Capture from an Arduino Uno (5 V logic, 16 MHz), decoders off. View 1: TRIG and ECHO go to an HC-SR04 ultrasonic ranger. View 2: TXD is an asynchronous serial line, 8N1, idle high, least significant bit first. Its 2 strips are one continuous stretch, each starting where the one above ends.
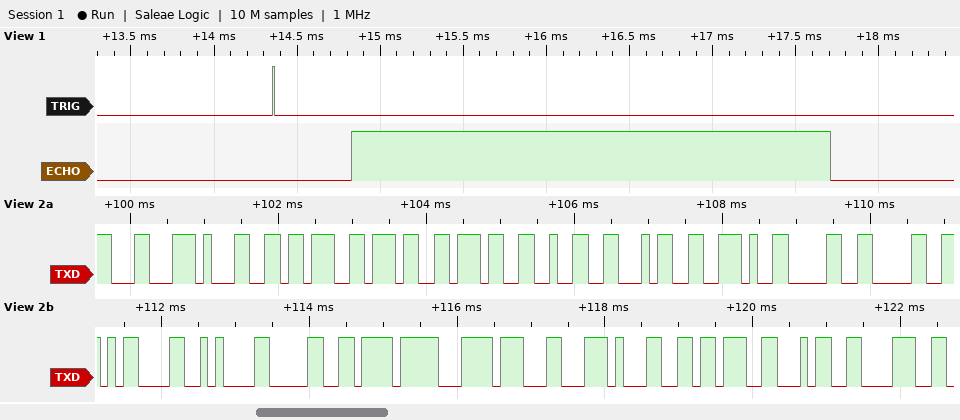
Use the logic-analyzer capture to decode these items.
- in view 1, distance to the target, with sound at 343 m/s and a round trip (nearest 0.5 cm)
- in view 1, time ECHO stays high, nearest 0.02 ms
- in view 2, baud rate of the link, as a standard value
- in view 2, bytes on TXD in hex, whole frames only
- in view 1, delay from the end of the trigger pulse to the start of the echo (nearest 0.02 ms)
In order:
49.5 cm
2.88 ms
9600 baud
8C 31 3B 37 37 32 34 2E 30 30 0D 0A 30 EF BC 8C 31 3B 34 38
0.46 ms
